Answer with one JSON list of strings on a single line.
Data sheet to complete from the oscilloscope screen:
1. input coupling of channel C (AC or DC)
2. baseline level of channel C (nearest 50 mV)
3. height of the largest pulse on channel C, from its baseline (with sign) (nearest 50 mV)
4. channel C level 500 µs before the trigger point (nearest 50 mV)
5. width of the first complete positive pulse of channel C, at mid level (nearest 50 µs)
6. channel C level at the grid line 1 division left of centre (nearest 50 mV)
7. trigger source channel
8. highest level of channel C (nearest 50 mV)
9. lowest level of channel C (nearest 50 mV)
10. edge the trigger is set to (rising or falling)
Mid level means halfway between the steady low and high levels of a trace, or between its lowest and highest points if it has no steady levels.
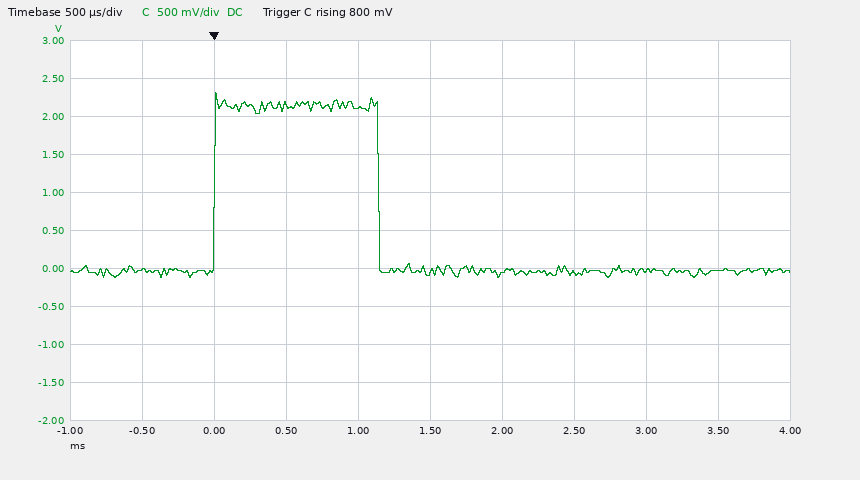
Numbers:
["DC", "-50 mV", "+2.35 V", "0 mV", "1.15 ms", "2.10 V", "channel C", "2.30 V", "-100 mV", "rising"]
